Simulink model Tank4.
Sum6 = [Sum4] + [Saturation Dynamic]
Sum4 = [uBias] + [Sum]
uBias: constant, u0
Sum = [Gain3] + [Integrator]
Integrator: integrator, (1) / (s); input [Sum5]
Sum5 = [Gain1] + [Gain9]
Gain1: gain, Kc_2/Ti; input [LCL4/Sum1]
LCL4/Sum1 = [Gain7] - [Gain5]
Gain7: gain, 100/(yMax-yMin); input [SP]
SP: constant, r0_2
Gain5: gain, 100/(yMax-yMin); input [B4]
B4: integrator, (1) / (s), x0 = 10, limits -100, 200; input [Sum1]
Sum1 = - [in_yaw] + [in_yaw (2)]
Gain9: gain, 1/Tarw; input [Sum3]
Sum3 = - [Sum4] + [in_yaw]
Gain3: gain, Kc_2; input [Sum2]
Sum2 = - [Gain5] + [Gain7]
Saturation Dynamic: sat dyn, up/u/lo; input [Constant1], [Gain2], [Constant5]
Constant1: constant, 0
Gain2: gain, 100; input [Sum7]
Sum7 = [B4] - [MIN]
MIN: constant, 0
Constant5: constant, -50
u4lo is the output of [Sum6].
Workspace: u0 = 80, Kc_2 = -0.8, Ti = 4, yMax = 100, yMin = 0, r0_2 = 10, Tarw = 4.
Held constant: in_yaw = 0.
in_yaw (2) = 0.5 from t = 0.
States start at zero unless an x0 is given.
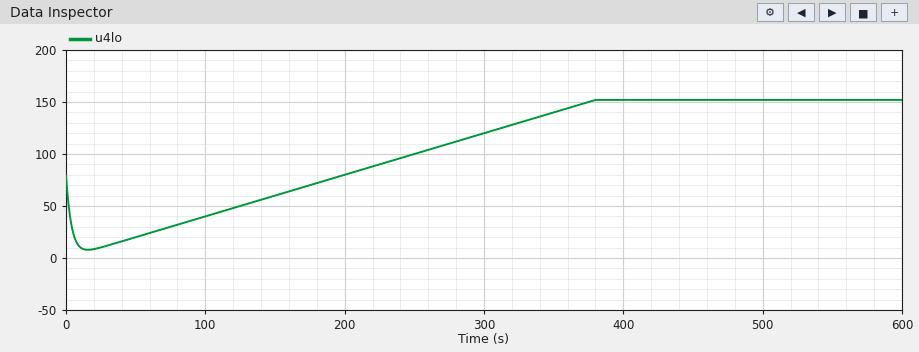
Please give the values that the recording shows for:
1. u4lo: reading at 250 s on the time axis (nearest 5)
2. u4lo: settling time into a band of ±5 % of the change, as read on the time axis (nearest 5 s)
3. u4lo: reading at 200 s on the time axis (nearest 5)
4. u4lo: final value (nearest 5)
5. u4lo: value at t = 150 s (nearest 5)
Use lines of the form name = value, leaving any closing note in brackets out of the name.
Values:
u4lo: reading at 250 s on the time axis = 100
u4lo: settling time into a band of ±5 % of the change, as read on the time axis = 370 s
u4lo: reading at 200 s on the time axis = 80
u4lo: final value = 150
u4lo: value at t = 150 s = 60
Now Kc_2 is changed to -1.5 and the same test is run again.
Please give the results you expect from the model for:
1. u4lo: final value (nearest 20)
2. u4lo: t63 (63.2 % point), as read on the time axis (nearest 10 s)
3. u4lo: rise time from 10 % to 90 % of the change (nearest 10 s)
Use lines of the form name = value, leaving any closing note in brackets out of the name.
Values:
u4lo: final value = 280
u4lo: t63 (63.2 % point), as read on the time axis = 280 s
u4lo: rise time from 10 % to 90 % of the change = 220 s
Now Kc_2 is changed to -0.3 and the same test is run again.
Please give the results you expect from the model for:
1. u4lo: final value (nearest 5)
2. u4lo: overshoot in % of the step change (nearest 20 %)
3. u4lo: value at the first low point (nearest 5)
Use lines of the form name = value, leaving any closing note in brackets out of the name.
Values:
u4lo: final value = 55
u4lo: overshoot in % of the step change = 240 %
u4lo: value at the first low point = 5
